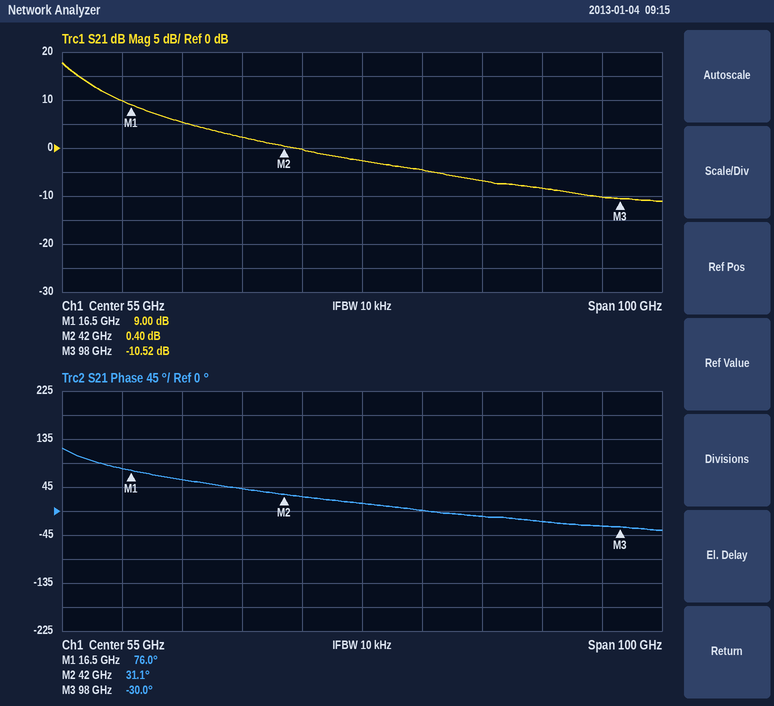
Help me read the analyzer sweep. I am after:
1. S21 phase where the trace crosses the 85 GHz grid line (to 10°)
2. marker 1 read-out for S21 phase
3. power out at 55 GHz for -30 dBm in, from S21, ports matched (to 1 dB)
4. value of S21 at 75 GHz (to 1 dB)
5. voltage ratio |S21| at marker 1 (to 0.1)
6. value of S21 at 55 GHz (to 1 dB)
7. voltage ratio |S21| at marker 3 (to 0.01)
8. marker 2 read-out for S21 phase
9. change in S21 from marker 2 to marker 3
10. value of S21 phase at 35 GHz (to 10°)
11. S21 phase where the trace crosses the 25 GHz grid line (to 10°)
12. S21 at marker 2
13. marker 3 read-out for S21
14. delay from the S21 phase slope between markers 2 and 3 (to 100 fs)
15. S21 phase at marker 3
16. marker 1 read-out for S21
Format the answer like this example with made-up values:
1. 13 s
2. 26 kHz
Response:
1. -20°
2. 76.0°
3. -33 dBm
4. -7 dB
5. 2.8
6. -3 dB
7. 0.30
8. 31.1°
9. -10.92 dB
10. 40°
11. 60°
12. 0.40 dB
13. -10.52 dB
14. 3.0 ps
15. -30.0°
16. 9.00 dB
